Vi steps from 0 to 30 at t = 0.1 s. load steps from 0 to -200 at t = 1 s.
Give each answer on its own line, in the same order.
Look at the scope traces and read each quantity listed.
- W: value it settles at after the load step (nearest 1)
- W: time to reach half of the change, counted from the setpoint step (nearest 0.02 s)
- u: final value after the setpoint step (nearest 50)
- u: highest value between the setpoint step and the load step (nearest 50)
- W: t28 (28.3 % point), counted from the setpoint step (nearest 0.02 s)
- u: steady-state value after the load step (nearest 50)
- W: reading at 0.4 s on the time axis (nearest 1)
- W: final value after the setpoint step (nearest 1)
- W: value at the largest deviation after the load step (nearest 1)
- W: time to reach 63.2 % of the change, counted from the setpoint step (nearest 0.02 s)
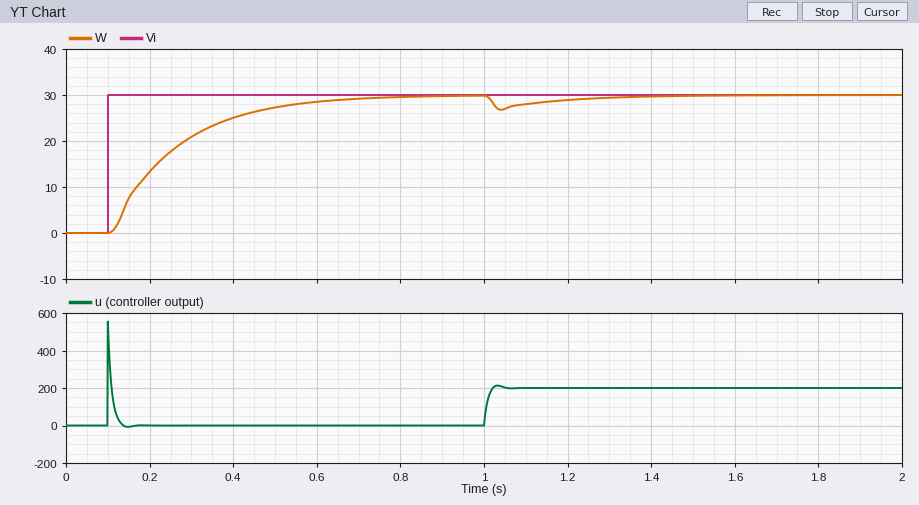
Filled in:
30
0.12 s
0
550
0.06 s
200
25
30
27
0.16 s
